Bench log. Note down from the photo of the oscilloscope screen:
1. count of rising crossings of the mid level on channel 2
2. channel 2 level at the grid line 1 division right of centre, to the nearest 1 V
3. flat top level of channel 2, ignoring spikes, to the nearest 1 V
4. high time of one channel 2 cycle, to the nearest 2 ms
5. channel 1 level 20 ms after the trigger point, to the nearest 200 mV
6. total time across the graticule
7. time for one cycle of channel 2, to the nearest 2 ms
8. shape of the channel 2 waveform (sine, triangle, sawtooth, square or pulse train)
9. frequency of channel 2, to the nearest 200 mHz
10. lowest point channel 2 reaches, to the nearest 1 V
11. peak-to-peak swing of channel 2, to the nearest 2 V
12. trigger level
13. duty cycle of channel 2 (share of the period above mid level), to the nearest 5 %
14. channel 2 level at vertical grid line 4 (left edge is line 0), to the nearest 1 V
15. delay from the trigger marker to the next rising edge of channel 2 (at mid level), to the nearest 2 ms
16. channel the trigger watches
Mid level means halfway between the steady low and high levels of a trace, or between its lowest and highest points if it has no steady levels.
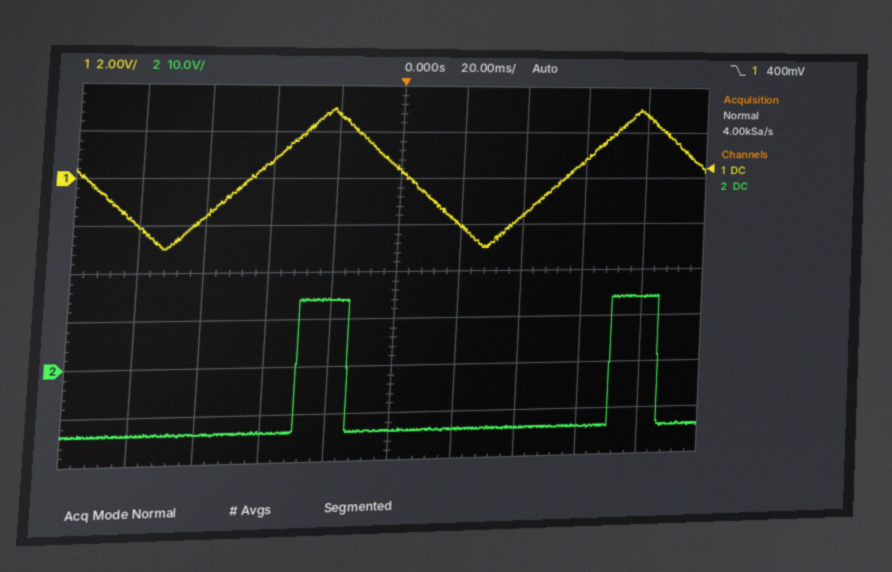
2
-14 V
14 V
16 ms
-2.0 V
200 ms
100 ms
pulse train
10.0 Hz
-14 V
28 V
400 mV
15 %
14 V
70 ms
channel 1
